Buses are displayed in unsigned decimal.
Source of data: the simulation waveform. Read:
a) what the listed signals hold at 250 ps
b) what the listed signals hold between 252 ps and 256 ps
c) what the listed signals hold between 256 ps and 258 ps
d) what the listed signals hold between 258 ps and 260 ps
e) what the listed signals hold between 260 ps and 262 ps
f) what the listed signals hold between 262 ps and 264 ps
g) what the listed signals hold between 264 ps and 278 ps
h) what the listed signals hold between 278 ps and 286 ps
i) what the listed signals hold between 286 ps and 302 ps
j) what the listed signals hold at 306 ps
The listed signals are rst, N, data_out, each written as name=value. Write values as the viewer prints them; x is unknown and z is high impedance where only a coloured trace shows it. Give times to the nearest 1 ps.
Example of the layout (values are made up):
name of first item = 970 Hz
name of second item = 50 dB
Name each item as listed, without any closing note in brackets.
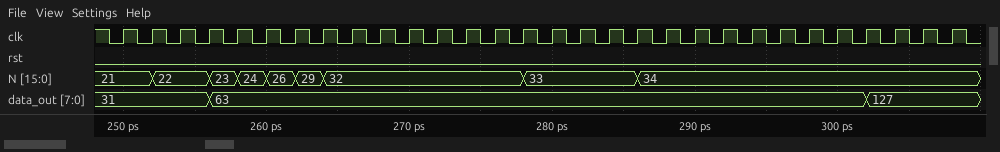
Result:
what the listed signals hold at 250 ps = rst=0, N=21, data_out=31
what the listed signals hold between 252 ps and 256 ps = rst=0, N=22, data_out=31
what the listed signals hold between 256 ps and 258 ps = rst=0, N=23, data_out=63
what the listed signals hold between 258 ps and 260 ps = rst=0, N=24, data_out=63
what the listed signals hold between 260 ps and 262 ps = rst=0, N=26, data_out=63
what the listed signals hold between 262 ps and 264 ps = rst=0, N=29, data_out=63
what the listed signals hold between 264 ps and 278 ps = rst=0, N=32, data_out=63
what the listed signals hold between 278 ps and 286 ps = rst=0, N=33, data_out=63
what the listed signals hold between 286 ps and 302 ps = rst=0, N=34, data_out=63
what the listed signals hold at 306 ps = rst=0, N=34, data_out=127
